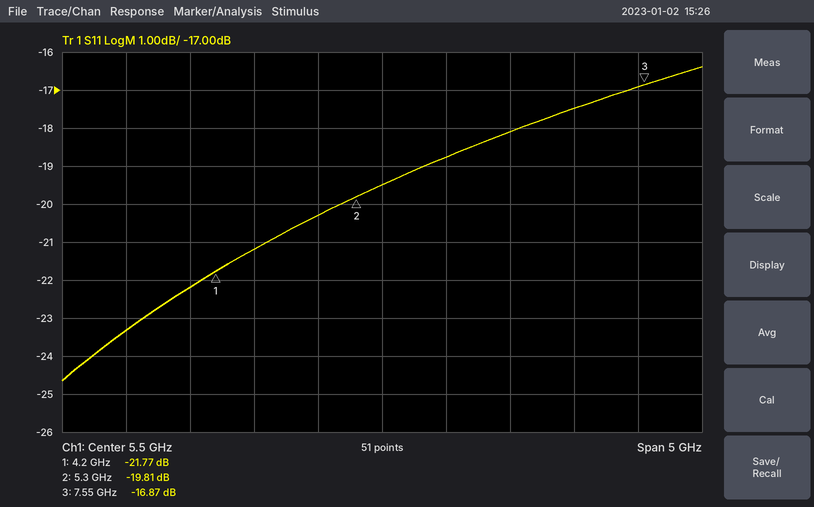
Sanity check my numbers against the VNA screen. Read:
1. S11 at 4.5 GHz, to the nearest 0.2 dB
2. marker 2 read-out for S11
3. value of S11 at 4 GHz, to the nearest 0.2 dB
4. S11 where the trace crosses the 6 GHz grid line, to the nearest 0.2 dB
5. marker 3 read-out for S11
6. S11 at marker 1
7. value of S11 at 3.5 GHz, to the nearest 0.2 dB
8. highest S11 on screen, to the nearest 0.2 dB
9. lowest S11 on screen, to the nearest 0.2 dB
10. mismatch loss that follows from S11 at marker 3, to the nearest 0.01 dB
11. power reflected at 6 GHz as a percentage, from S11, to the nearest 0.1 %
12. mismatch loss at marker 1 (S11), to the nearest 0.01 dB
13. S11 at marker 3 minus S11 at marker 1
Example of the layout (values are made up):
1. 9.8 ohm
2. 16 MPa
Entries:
1. -21.2 dB
2. -19.81 dB
3. -22.2 dB
4. -18.8 dB
5. -16.87 dB
6. -21.77 dB
7. -23.4 dB
8. -16.4 dB
9. -24.6 dB
10. 0.09 dB
11. 1.3 %
12. 0.03 dB
13. 4.90 dB
